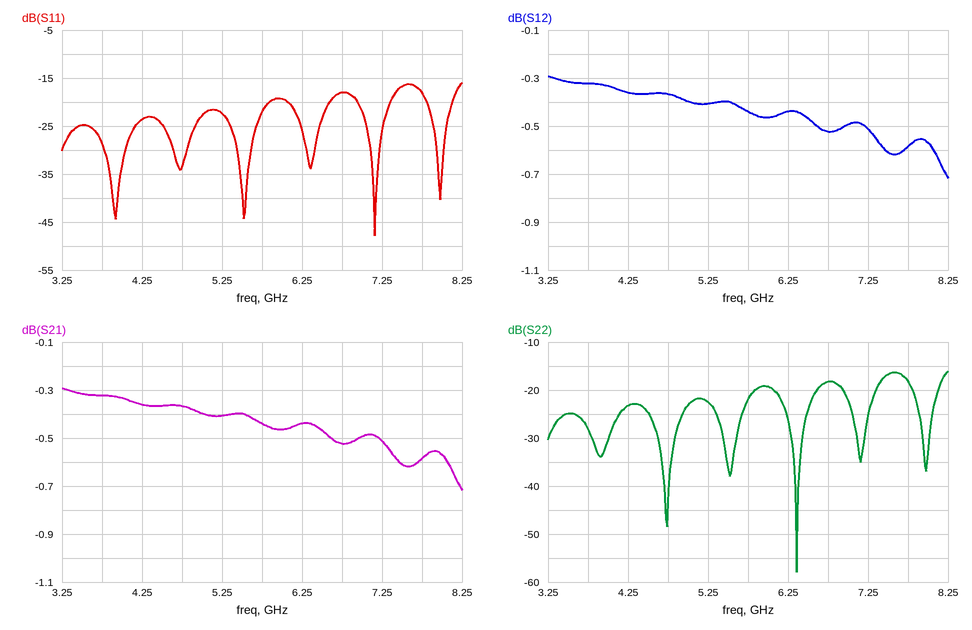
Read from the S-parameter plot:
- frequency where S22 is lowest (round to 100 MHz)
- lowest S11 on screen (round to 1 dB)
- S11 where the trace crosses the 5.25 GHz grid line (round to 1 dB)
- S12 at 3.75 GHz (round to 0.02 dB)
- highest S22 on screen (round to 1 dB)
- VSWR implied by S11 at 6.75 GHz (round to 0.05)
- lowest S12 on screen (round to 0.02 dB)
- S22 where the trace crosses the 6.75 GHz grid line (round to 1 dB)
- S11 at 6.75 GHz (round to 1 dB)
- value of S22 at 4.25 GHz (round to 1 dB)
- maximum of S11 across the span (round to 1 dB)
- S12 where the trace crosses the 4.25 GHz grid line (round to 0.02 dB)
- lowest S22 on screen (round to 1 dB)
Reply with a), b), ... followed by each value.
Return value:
a) 6.4 GHz
b) -48 dB
c) -22 dB
d) -0.32 dB
e) -16 dB
f) 1.30
g) -0.72 dB
h) -18 dB
i) -18 dB
j) -23 dB
k) -16 dB
l) -0.36 dB
m) -58 dB
